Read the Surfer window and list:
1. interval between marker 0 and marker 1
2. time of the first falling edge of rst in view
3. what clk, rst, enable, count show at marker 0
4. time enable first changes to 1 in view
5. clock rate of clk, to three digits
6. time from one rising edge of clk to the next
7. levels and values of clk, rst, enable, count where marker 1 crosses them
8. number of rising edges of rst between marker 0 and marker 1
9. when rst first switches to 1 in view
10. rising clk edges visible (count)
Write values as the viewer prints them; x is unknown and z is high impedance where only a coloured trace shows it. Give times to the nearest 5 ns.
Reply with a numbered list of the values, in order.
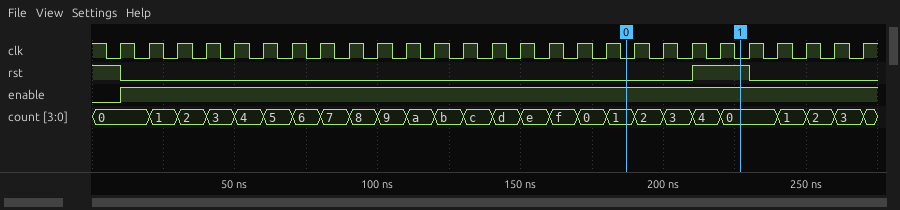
1. 40 ns
2. 10 ns
3. clk=0, rst=0, enable=1, count=1
4. 10 ns
5. 100 MHz
6. 10 ns
7. clk=0, rst=1, enable=1, count=0
8. 1
9. 210 ns
10. 27
